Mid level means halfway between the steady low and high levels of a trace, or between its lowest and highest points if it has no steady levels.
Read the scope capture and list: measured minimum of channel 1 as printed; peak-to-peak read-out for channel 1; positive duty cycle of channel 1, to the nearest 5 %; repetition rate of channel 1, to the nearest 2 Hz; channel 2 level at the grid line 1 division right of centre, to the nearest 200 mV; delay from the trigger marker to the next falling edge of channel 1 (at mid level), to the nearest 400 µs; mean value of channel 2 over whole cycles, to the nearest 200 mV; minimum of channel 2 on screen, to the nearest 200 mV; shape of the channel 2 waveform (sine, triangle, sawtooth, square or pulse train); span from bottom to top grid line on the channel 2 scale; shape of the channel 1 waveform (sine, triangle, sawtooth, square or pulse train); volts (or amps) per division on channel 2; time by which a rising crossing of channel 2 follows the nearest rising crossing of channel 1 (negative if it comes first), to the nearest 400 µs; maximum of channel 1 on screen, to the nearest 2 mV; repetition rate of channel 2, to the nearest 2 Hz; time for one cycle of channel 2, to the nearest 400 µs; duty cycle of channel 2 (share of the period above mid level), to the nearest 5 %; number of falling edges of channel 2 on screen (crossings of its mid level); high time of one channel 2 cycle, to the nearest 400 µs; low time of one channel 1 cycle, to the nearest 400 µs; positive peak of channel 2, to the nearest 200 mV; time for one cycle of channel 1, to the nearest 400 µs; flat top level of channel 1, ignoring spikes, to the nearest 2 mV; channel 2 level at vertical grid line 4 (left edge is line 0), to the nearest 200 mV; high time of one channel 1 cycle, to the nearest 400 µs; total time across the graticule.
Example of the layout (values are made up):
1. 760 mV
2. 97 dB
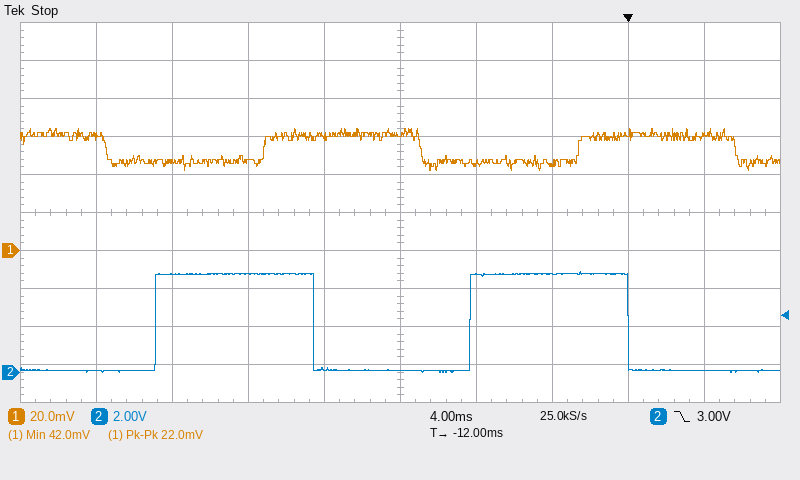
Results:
1. 42.0 mV
2. 22.0 mV
3. 50 %
4. 60 Hz
5. 5.2 V
6. 5.6 ms
7. 2.6 V
8. 0.0 V
9. square
10. 20 V
11. square
12. 2 V
13. -5.6 ms
14. 64 mV
15. 60 Hz
16. 16.4 ms
17. 50 %
18. 2
19. 8.4 ms
20. 8.4 ms
21. 5.2 V
22. 16.4 ms
23. 60 mV
24. 200 mV
25. 8.4 ms
26. 40 ms
